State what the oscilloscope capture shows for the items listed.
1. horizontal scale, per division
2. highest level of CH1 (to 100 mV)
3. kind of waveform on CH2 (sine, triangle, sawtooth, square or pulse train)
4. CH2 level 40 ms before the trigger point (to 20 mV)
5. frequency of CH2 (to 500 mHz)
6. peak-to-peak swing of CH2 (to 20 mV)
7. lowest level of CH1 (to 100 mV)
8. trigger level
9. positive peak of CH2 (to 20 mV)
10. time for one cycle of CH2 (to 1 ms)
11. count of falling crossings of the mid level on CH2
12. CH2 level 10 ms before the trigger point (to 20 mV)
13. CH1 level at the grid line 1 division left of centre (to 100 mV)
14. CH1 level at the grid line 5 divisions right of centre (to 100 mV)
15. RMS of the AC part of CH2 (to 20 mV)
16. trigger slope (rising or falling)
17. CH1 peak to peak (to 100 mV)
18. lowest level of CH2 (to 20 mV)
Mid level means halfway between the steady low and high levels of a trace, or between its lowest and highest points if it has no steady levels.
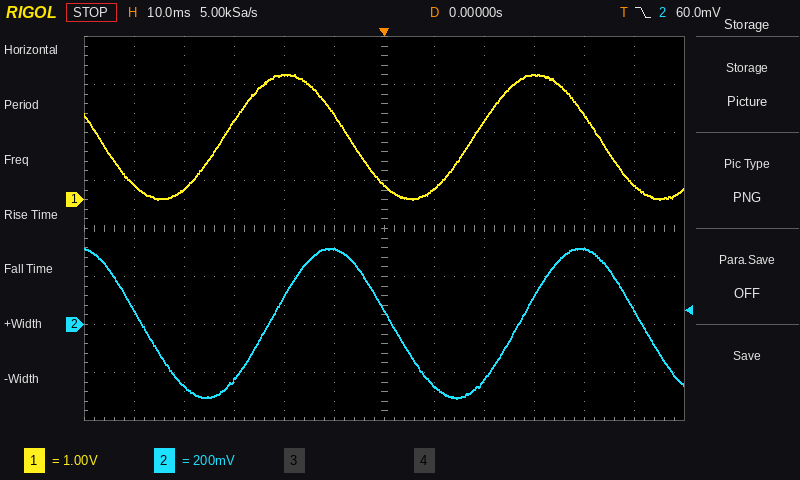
10 ms
2.6 V
sine
-260 mV
20.0 Hz
620 mV
0.0 V
60.0 mV
320 mV
50 ms
3
320 mV
1.8 V
300 mV
220 mV
falling
2.6 V
-300 mV
